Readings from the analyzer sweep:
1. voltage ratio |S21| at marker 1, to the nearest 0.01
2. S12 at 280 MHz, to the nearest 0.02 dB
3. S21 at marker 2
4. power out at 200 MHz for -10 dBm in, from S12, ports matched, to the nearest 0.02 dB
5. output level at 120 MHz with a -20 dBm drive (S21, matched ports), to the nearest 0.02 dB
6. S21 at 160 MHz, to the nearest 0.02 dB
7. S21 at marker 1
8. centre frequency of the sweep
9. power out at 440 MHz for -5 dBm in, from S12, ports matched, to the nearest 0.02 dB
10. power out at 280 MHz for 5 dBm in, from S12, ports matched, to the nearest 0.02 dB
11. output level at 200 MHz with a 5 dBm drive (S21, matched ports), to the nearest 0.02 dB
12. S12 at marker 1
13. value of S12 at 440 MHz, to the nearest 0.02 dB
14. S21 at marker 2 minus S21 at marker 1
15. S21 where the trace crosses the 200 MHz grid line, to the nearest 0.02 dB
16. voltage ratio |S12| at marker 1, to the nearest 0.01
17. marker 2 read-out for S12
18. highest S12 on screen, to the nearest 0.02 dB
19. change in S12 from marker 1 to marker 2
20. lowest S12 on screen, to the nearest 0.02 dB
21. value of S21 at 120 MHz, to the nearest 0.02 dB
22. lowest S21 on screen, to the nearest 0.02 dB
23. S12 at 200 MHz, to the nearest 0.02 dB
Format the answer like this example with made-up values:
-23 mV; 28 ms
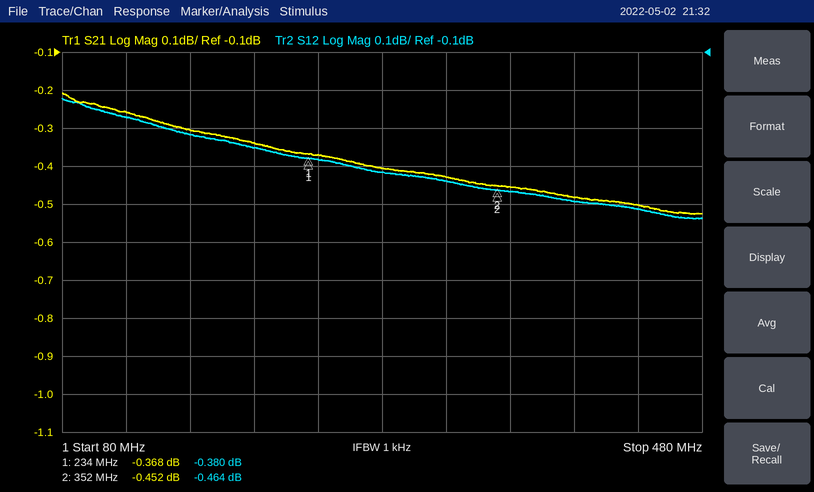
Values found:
0.96; -0.42 dB; -0.452 dB; -10.36 dBm; -20.26 dBm; -0.30 dB; -0.368 dB; 280 MHz; -5.52 dBm; 4.58 dBm; 4.66 dBm; -0.380 dB; -0.52 dB; -0.084 dB; -0.34 dB; 0.96; -0.464 dB; -0.22 dB; -0.084 dB; -0.54 dB; -0.26 dB; -0.52 dB; -0.36 dB
